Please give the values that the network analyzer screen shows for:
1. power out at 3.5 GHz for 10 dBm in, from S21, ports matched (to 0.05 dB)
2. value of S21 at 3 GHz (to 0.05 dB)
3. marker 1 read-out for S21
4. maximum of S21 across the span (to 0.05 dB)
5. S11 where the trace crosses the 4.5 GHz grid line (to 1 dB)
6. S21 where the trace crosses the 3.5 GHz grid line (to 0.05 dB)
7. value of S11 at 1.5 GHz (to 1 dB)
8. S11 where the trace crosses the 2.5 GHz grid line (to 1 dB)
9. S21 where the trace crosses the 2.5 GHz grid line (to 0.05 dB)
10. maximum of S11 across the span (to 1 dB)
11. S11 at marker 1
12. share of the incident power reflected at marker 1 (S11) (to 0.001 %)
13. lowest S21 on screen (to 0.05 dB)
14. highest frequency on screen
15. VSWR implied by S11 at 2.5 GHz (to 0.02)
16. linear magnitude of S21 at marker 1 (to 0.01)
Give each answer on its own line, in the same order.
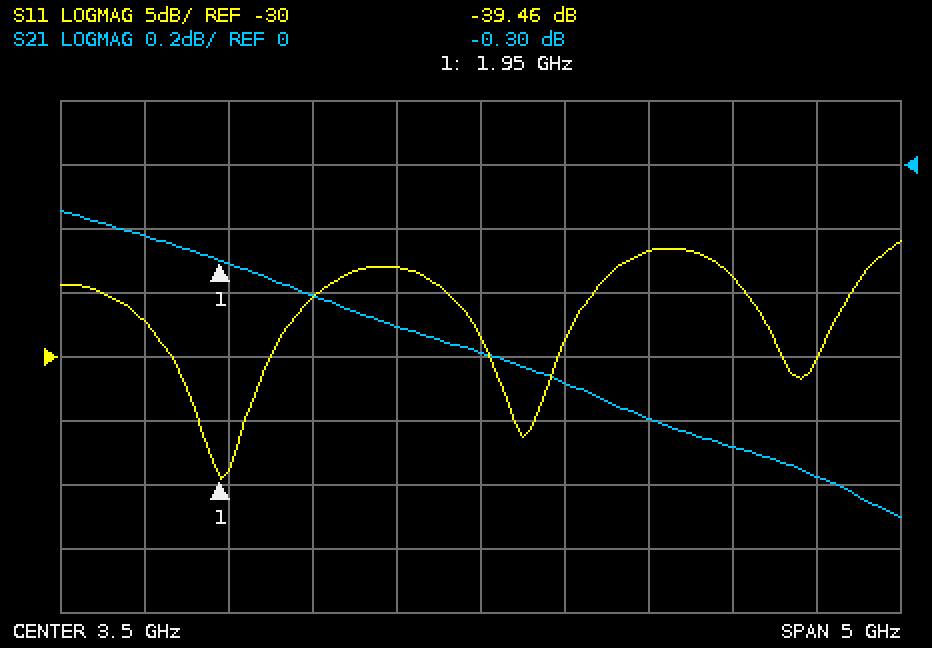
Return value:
9.40 dBm
-0.50 dB
-0.30 dB
-0.15 dB
-22 dB
-0.60 dB
-27 dB
-25 dB
-0.40 dB
-21 dB
-39.46 dB
0.011 %
-1.10 dB
6 GHz
1.12
0.97
